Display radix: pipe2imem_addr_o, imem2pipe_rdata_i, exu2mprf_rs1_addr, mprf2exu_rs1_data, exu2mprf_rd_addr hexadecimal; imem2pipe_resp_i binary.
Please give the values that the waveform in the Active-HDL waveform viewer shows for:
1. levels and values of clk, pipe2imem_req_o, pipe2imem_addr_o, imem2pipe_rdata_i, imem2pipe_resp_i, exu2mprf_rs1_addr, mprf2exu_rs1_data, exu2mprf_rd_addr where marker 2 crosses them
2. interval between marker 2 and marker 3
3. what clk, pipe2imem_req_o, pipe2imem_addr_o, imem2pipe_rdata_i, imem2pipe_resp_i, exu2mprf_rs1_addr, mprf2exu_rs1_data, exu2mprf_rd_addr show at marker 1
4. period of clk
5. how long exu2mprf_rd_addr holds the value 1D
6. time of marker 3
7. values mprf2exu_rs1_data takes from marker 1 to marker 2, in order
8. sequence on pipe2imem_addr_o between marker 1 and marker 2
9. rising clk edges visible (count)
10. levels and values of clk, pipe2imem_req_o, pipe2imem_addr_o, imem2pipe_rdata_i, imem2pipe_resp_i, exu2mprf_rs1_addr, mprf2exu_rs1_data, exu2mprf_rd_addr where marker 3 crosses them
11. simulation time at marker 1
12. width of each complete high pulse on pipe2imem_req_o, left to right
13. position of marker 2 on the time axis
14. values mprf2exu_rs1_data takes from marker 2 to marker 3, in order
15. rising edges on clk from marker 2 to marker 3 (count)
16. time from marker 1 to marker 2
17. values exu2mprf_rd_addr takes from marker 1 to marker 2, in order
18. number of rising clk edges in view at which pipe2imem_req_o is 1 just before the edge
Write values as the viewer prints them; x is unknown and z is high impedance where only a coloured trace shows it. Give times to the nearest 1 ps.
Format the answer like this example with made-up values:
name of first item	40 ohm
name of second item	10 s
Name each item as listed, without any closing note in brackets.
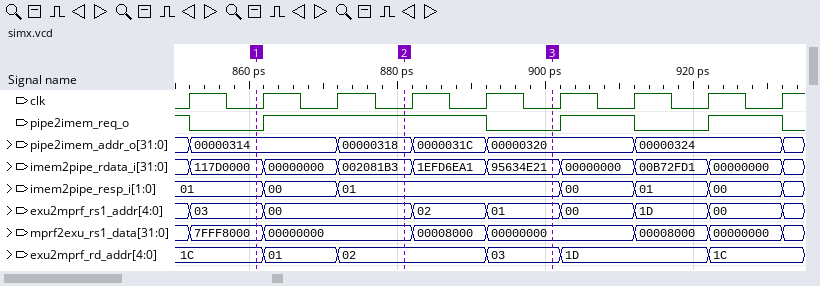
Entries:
levels and values of clk, pipe2imem_req_o, pipe2imem_addr_o, imem2pipe_rdata_i, imem2pipe_resp_i, exu2mprf_rs1_addr, mprf2exu_rs1_data, exu2mprf_rd_addr where marker 2 crosses them	clk=0, pipe2imem_req_o=1, pipe2imem_addr_o=00000318, imem2pipe_rdata_i=002081B3, imem2pipe_resp_i=01, exu2mprf_rs1_addr=00, mprf2exu_rs1_data=00000000, exu2mprf_rd_addr=02
interval between marker 2 and marker 3	20 ps
what clk, pipe2imem_req_o, pipe2imem_addr_o, imem2pipe_rdata_i, imem2pipe_resp_i, exu2mprf_rs1_addr, mprf2exu_rs1_data, exu2mprf_rd_addr show at marker 1	clk=0, pipe2imem_req_o=0, pipe2imem_addr_o=00000314, imem2pipe_rdata_i=117D0000, imem2pipe_resp_i=01, exu2mprf_rs1_addr=03, mprf2exu_rs1_data=7FFF8000, exu2mprf_rd_addr=1C
period of clk	10 ps
how long exu2mprf_rd_addr holds the value 1D	20 ps
time of marker 3	901 ps
values mprf2exu_rs1_data takes from marker 1 to marker 2, in order	7FFF8000, 00000000
sequence on pipe2imem_addr_o between marker 1 and marker 2	00000314, 00000318
rising clk edges visible	9
levels and values of clk, pipe2imem_req_o, pipe2imem_addr_o, imem2pipe_rdata_i, imem2pipe_resp_i, exu2mprf_rs1_addr, mprf2exu_rs1_data, exu2mprf_rd_addr where marker 3 crosses them	clk=0, pipe2imem_req_o=0, pipe2imem_addr_o=00000320, imem2pipe_rdata_i=95634E21, imem2pipe_resp_i=01, exu2mprf_rs1_addr=01, mprf2exu_rs1_data=00000000, exu2mprf_rd_addr=03
simulation time at marker 1	861 ps
width of each complete high pulse on pipe2imem_req_o, left to right	30 ps, 10 ps, 10 ps
position of marker 2 on the time axis	881 ps
values mprf2exu_rs1_data takes from marker 2 to marker 3, in order	00000000, 00008000, 00000000
rising edges on clk from marker 2 to marker 3	2
time from marker 1 to marker 2	20 ps
values exu2mprf_rd_addr takes from marker 1 to marker 2, in order	1C, 01, 02
number of rising clk edges in view at which pipe2imem_req_o is 1 just before the edge	6
